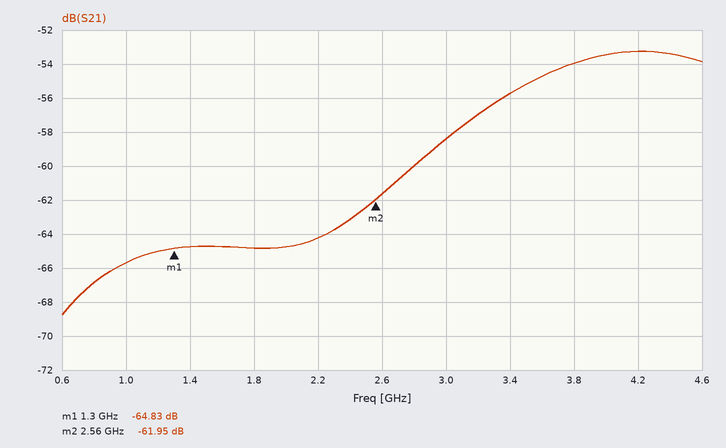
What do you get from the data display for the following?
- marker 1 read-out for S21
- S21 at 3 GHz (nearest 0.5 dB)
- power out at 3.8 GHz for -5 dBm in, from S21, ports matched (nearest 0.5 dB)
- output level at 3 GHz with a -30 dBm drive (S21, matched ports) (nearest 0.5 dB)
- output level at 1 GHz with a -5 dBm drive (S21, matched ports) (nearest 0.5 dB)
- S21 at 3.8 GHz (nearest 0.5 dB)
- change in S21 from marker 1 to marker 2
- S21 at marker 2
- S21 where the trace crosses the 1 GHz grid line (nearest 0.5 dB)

-64.83 dB
-58.5 dB
-59.0 dBm
-88.5 dBm
-70.5 dBm
-54.0 dB
2.88 dB
-61.95 dB
-65.5 dB
